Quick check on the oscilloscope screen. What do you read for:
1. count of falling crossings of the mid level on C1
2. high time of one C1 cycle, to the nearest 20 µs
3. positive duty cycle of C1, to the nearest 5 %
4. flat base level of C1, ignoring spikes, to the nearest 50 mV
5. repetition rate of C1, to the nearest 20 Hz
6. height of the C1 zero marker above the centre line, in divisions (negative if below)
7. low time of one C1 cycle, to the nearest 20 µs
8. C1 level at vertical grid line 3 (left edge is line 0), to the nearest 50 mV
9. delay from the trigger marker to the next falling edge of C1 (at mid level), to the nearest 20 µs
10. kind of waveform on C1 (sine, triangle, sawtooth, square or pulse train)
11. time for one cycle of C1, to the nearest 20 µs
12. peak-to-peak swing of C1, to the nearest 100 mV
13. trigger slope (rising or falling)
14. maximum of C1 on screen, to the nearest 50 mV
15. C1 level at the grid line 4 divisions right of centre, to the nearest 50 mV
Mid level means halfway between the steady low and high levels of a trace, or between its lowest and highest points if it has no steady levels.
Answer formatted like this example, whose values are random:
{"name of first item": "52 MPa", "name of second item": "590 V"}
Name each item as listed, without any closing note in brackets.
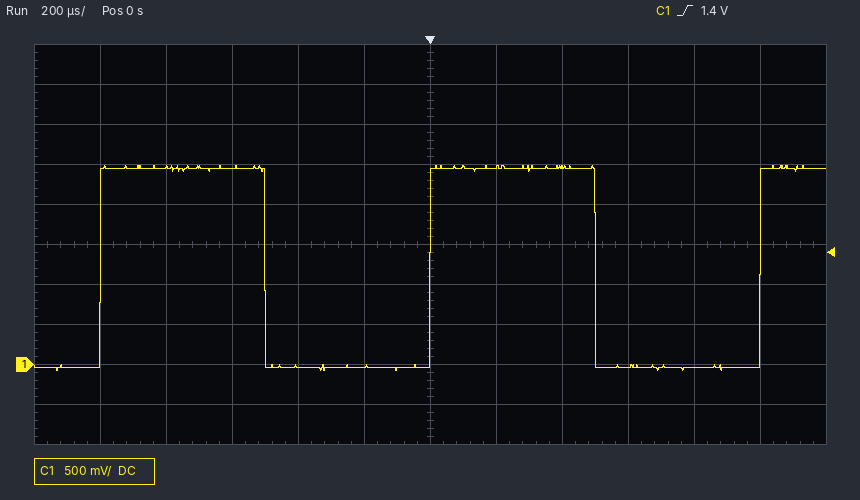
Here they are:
{"count of falling crossings of the mid level on C1": "2", "high time of one C1 cycle, to the nearest 20 µs": "500 µs", "positive duty cycle of C1, to the nearest 5 %": "50 %", "flat base level of C1, ignoring spikes, to the nearest 50 mV": "-50 mV", "repetition rate of C1, to the nearest 20 Hz": "1.00 kHz", "height of the C1 zero marker above the centre line, in divisions": "-3.0 div", "low time of one C1 cycle, to the nearest 20 µs": "500 µs", "C1 level at vertical grid line 3 (left edge is line 0), to the nearest 50 mV": "2.45 V", "delay from the trigger marker to the next falling edge of C1 (at mid level), to the nearest 20 µs": "500 µs", "kind of waveform on C1": "square", "time for one cycle of C1, to the nearest 20 µs": "1.00 ms", "peak-to-peak swing of C1, to the nearest 100 mV": "2.60 V", "trigger slope": "rising", "maximum of C1 on screen, to the nearest 50 mV": "2.50 V", "C1 level at the grid line 4 divisions right of centre, to the nearest 50 mV": "-50 mV"}
